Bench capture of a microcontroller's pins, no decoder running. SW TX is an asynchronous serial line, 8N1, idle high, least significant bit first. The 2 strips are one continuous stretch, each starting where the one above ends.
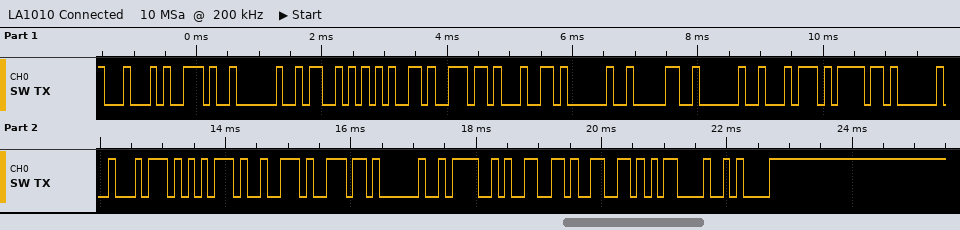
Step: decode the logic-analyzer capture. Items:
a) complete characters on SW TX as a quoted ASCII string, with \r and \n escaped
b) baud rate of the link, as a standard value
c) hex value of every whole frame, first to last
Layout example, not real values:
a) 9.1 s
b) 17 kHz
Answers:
a) "D. Send 0 to turn Off\r\n"
b) 9600 baud
c) 44 2E 20 53 65 6E 64 20 30 20 74 6F 20 74 75 72 6E 20 4F 66 66 0D 0A
